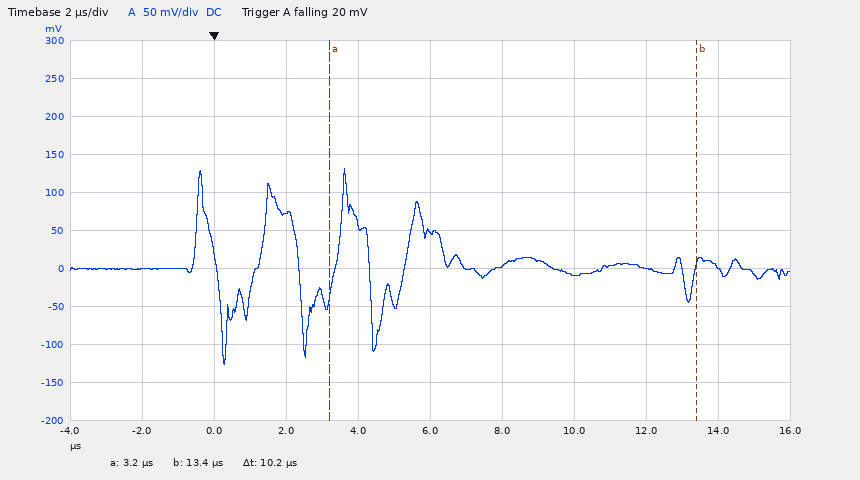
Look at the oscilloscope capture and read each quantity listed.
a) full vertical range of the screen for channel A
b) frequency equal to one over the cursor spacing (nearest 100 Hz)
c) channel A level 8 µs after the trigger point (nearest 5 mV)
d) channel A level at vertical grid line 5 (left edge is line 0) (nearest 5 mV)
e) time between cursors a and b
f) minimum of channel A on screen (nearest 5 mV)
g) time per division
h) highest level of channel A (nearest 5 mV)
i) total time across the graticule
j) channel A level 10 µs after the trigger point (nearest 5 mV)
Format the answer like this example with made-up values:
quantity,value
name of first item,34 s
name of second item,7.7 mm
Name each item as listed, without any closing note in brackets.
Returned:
quantity,value
full vertical range of the screen for channel A,500 mV
frequency equal to one over the cursor spacing,98.0 kHz
channel A level 8 µs after the trigger point,5 mV
channel A level at vertical grid line 5 (left edge is line 0),50 mV
time between cursors a and b,10.2 µs
minimum of channel A on screen,-125 mV
time per division,2 µs
highest level of channel A,130 mV
total time across the graticule,20 µs
channel A level 10 µs after the trigger point,-10 mV
